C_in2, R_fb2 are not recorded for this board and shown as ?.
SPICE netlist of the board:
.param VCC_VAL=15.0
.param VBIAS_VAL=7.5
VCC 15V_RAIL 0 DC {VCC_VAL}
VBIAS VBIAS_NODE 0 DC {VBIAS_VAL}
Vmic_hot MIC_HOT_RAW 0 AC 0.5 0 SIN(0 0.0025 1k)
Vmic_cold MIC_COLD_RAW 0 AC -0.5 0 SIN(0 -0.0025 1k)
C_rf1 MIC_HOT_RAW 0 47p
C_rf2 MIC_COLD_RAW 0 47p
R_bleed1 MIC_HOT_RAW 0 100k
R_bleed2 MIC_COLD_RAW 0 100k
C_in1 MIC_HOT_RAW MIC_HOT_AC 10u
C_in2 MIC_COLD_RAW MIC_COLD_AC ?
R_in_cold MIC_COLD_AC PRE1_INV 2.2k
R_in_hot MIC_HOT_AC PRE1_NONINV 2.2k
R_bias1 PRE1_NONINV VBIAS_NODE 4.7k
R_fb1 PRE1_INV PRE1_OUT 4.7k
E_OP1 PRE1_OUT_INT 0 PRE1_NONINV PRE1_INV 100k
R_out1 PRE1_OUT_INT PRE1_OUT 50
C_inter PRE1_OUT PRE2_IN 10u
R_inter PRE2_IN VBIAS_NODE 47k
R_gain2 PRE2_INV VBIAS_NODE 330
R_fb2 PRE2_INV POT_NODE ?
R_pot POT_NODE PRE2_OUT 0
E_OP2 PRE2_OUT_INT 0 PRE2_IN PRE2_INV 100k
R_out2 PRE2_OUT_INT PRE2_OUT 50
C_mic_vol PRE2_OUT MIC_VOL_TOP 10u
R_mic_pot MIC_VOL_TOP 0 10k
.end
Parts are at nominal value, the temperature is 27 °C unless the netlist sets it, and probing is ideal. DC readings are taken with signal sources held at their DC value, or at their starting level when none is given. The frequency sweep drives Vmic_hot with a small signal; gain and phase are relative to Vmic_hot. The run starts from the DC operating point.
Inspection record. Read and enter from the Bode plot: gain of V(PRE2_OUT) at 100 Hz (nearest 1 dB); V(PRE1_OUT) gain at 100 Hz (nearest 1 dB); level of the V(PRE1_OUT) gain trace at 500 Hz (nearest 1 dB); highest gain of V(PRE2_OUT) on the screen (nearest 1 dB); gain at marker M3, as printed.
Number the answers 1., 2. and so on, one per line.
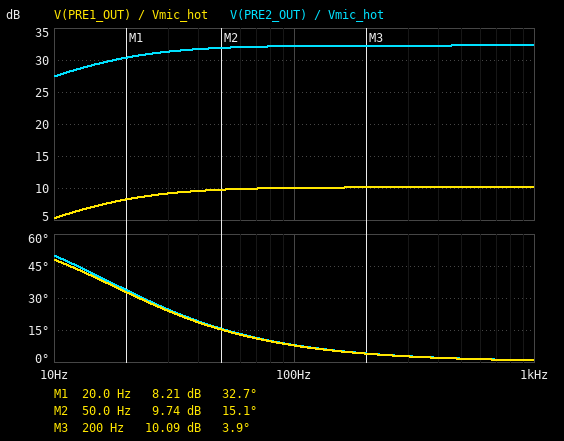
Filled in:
1. 32 dB
2. 10 dB
3. 10 dB
4. 32 dB
5. 10.09 dB
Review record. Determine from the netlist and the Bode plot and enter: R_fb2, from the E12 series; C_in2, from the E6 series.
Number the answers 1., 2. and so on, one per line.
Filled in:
1. 3.9 kΩ
2. 4.7 µF
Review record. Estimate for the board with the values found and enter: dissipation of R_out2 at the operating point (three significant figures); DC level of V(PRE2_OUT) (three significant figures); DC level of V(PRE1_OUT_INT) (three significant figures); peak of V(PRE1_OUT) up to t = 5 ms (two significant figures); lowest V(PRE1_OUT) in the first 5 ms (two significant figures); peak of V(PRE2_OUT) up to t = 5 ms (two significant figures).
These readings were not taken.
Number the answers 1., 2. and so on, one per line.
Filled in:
1. 147 nW
2. 7.50 V
3. 7.50 V
4. 7.5 V
5. 7.5 V
6. 7.6 V
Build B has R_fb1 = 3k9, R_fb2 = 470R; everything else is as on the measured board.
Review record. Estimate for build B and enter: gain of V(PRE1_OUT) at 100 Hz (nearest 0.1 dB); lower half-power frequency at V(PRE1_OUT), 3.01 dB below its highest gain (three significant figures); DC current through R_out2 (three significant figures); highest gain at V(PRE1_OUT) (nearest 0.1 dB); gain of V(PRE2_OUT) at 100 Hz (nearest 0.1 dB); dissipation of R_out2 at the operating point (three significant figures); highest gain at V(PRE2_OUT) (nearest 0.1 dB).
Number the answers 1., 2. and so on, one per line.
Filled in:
1. 8.8 dB
2. 14.4 Hz
3. 247 µA
4. 8.9 dB
5. 16.5 dB
6. 3.06 µW
7. 16.6 dB
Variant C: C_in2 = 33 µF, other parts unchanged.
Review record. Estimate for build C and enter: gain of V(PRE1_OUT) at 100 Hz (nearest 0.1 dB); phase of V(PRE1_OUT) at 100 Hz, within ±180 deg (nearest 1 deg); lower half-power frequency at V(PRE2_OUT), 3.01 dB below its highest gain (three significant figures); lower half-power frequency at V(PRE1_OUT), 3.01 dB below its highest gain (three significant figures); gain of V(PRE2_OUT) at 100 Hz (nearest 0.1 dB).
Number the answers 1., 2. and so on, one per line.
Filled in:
1. 10.1 dB
2. 2 deg
3. 3.15 Hz
4. 3.12 Hz
5. 32.3 dB
